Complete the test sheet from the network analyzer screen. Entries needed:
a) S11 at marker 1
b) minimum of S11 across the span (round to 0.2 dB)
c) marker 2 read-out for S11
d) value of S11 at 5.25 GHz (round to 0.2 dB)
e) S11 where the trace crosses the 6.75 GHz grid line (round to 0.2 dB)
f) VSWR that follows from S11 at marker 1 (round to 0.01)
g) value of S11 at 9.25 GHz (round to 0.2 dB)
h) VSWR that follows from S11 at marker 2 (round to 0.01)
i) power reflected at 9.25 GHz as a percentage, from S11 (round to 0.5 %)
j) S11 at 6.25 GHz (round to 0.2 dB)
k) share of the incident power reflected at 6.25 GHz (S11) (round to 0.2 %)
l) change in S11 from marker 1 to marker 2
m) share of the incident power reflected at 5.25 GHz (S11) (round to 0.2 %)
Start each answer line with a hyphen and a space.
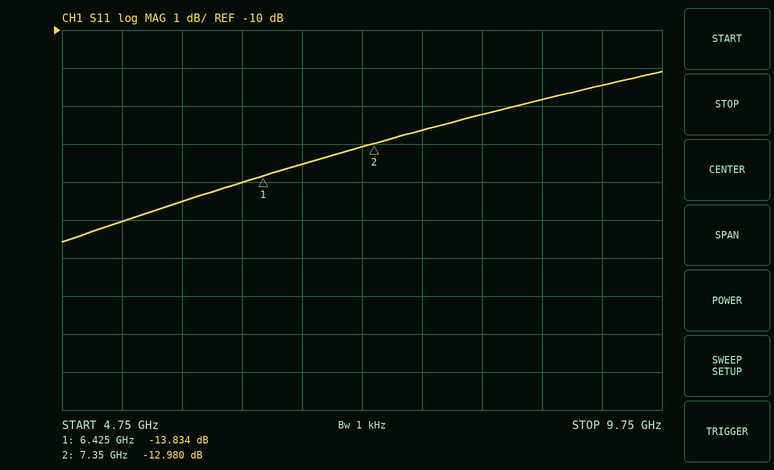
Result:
- -13.834 dB
- -15.6 dB
- -12.980 dB
- -15.0 dB
- -13.6 dB
- 1.51
- -11.4 dB
- 1.58
- 7.0 %
- -14.0 dB
- 4.0 %
- 0.854 dB
- 3.2 %
